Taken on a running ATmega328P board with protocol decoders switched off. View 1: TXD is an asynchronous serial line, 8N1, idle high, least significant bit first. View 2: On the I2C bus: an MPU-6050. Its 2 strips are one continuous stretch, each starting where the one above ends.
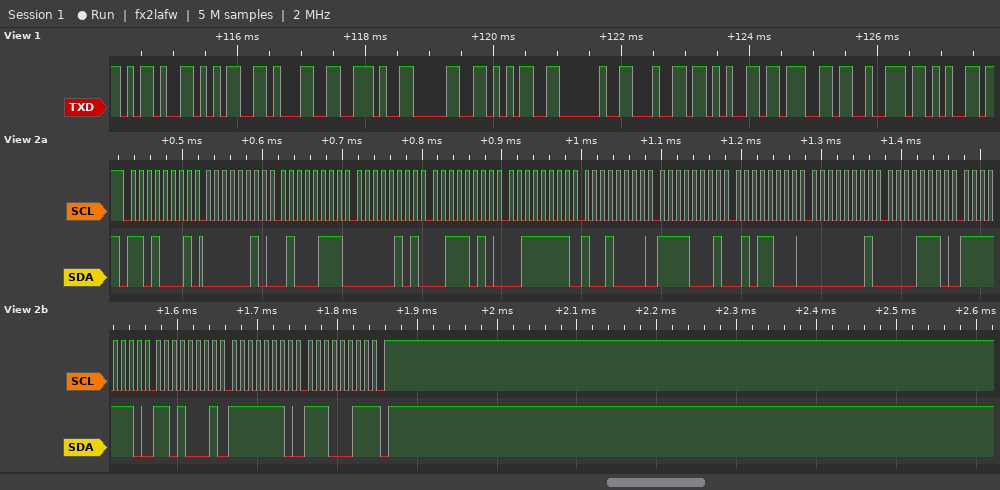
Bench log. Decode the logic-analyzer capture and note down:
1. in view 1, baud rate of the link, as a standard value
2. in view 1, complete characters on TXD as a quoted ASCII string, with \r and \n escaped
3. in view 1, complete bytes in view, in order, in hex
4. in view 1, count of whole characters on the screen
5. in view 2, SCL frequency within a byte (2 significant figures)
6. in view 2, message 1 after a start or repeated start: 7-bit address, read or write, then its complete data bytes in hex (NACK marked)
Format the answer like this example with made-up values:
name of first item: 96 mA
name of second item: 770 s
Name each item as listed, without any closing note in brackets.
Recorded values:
in view 1, baud rate of the link, as a standard value: 9600 baud
in view 1, complete characters on TXD as a quoted ASCII string, with \r and \n escaped: "-51.05 degre"
in view 1, complete bytes in view, in order, in hex: 2D 35 31 2E 30 35 20 64 65 67 72 65
in view 1, count of whole characters on the screen: 12
in view 2, SCL frequency within a byte: 100 kHz
in view 2, message 1 after a start or repeated start: 7-bit address, read or write, then its complete data bytes in hex: 0x68 read: 02 47 05 3A 3F 90 F1 58 01 0E FE D1 FE E3 NACK
